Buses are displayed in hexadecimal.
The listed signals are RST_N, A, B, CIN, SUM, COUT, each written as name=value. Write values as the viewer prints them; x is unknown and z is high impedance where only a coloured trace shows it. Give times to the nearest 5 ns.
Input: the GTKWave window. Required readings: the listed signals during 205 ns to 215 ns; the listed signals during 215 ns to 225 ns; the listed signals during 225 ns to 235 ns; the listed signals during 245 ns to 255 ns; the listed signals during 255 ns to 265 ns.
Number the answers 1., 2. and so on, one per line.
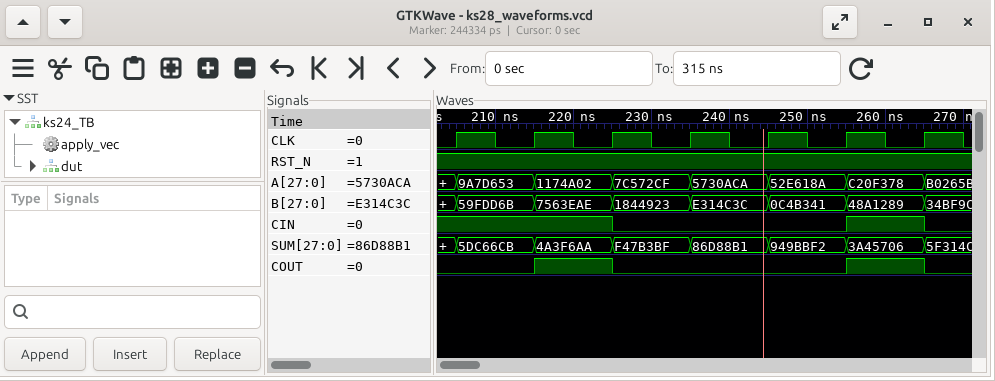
1. RST_N=1, A=9A7D653, B=59FDD6B, CIN=1, SUM=5DC66CB, COUT=0
2. RST_N=1, A=1174A02, B=7563EAE, CIN=1, SUM=4A3F6AA, COUT=1
3. RST_N=1, A=7C572CF, B=1844923, CIN=0, SUM=F47B3BF, COUT=0
4. RST_N=1, A=52E618A, B=0C4B341, CIN=0, SUM=949BBF2, COUT=0
5. RST_N=1, A=C20F378, B=48A1289, CIN=1, SUM=3A45706, COUT=1
